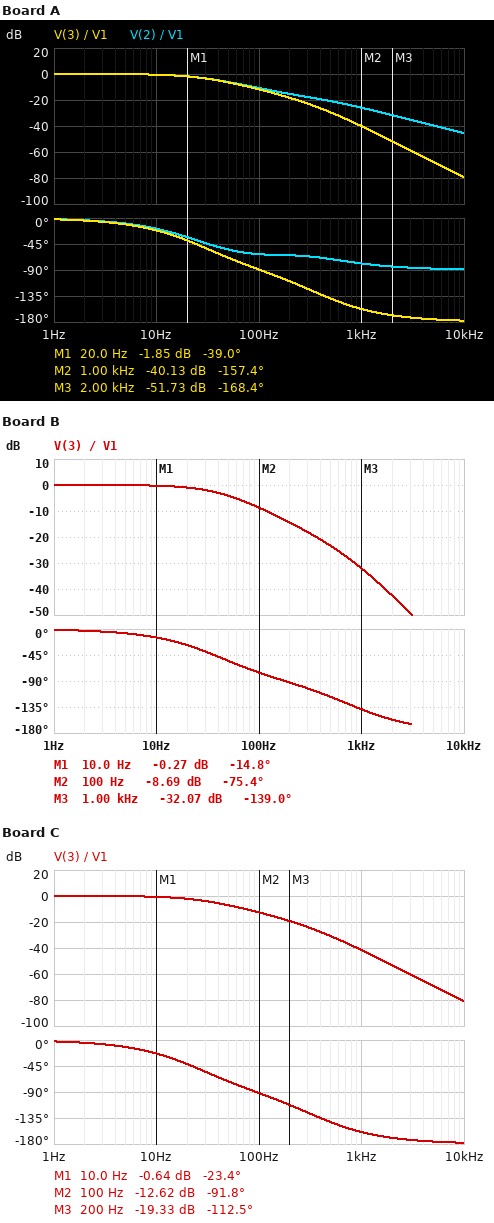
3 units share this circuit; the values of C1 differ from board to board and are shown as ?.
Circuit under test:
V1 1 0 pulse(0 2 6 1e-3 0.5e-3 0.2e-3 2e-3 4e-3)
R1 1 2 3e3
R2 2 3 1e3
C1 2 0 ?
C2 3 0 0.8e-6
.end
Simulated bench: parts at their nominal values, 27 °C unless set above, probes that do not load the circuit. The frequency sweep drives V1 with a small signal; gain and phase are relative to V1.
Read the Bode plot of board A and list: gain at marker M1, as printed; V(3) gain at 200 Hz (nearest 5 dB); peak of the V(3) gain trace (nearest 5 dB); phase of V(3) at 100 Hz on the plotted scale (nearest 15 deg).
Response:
-1.85 dB
-20 dB
0 dB
-90 deg
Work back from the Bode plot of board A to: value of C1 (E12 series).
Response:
1 µF
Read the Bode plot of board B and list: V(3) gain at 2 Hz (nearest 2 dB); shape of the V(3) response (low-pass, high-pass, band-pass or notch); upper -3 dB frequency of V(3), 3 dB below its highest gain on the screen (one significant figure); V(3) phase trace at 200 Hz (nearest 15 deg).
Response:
0 dB
low-pass
40 Hz
-90 deg
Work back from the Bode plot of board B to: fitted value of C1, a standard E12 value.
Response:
330 nF
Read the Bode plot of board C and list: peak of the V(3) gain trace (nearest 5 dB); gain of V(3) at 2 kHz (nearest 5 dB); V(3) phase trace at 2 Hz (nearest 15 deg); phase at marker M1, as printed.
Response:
0 dB
-55 dB
0 deg
-23.4 deg
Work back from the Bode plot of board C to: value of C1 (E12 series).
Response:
1.2 µF
